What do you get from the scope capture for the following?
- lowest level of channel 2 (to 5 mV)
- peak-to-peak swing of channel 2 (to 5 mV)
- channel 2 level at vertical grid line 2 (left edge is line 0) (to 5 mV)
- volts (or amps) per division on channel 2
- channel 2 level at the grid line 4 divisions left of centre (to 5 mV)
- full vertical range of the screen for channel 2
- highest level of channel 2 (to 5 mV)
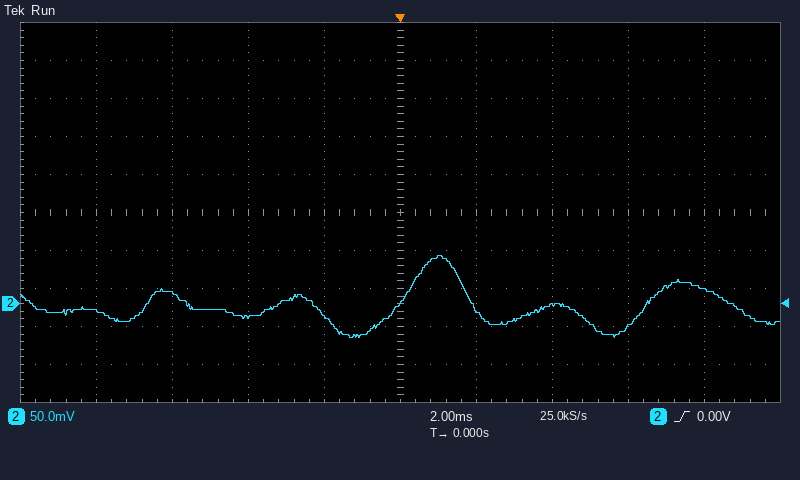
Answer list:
-45 mV
110 mV
15 mV
50 mV
-10 mV
500 mV
65 mV
